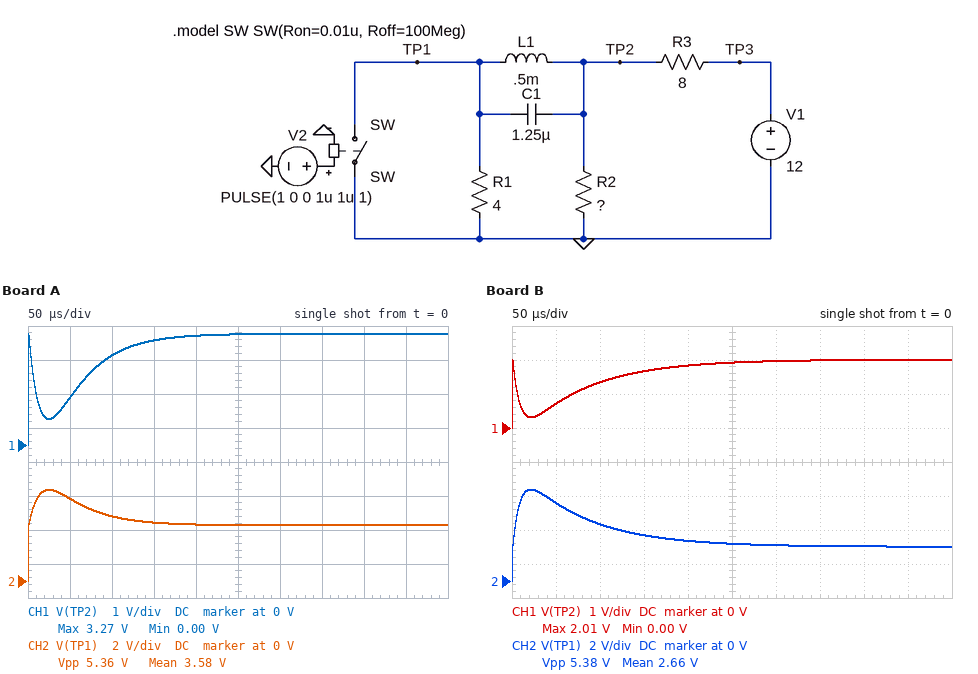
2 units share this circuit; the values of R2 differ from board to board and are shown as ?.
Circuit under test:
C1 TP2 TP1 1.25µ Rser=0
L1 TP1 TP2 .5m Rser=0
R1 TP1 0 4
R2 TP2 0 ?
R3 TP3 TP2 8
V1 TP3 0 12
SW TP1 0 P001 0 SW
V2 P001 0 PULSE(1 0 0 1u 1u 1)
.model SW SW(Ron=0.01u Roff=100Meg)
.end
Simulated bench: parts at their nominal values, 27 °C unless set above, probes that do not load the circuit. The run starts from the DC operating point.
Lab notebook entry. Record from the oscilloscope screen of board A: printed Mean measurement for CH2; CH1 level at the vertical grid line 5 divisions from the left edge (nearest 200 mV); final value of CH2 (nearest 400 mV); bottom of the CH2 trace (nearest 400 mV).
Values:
3.58 V
3.2 V
3.2 V
0 V
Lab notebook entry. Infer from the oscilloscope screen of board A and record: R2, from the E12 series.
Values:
12 Ω
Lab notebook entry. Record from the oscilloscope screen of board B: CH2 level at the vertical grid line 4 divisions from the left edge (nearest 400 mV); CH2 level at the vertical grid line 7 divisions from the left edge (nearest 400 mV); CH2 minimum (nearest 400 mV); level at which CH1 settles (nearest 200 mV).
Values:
2.4 V
2.0 V
0 V
2.0 V
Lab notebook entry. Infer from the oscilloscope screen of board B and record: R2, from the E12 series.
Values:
2.7 Ω
